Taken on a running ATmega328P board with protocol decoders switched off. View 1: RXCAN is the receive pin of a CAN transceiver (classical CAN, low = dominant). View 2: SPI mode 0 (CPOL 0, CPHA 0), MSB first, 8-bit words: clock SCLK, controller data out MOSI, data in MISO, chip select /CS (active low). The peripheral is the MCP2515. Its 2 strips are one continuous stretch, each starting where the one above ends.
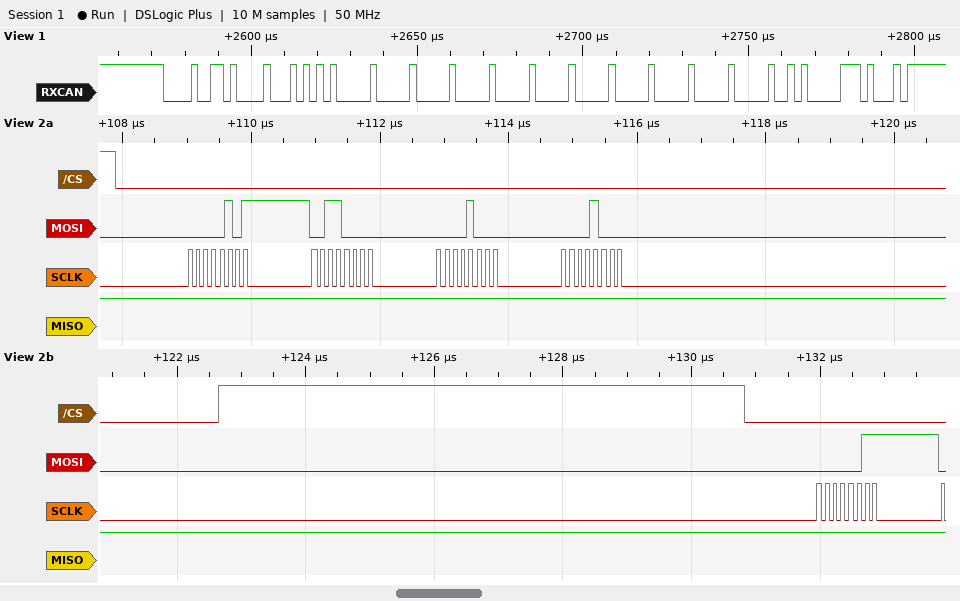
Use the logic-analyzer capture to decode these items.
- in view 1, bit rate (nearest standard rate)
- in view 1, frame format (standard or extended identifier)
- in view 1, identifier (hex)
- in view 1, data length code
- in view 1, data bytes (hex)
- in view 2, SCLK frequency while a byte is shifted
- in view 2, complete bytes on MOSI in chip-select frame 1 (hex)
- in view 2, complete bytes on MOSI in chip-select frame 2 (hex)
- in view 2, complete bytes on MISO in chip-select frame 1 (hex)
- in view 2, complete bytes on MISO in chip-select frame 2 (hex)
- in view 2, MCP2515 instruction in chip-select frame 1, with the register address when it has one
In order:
500 kbit/s
standard
0x09A
8
AA 00 00 00 00 00 00 00
8 MHz
05 30 08 08
03
FF FF FF FF
FF
BIT MODIFY 0x30
